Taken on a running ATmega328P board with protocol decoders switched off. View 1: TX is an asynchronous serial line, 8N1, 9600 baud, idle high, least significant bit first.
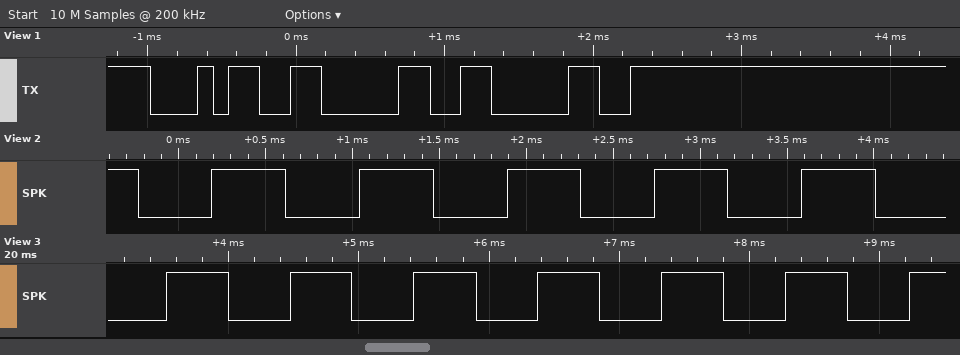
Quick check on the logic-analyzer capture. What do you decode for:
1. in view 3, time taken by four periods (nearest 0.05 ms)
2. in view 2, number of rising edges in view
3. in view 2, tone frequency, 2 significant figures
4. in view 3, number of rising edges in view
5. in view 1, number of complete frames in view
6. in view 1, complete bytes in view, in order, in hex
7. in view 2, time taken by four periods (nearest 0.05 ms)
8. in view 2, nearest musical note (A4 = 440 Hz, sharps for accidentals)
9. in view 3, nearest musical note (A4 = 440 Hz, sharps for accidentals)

3.80 ms
5
1.2 kHz
7
3
34 30 30
3.40 ms
D6
C6
